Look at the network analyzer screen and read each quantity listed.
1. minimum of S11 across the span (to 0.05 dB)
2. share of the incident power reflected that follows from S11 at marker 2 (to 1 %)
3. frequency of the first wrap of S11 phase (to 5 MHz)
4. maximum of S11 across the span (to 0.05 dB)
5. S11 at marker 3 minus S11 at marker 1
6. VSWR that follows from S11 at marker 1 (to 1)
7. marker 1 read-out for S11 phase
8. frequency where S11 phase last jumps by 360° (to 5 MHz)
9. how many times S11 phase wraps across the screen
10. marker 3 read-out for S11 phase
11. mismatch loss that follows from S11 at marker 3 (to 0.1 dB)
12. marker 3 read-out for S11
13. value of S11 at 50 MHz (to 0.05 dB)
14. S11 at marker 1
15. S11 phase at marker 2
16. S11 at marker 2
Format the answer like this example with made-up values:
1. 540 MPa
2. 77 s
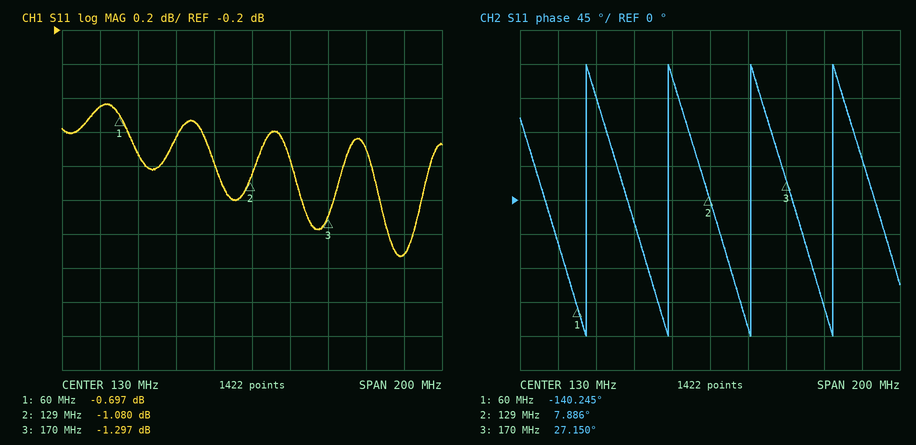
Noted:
1. -1.55 dB
2. 78 %
3. 65 MHz
4. -0.65 dB
5. -0.600 dB
6. 25
7. -140.245°
8. 195 MHz
9. 4
10. 27.150°
11. 5.9 dB
12. -1.297 dB
13. -0.65 dB
14. -0.697 dB
15. 7.886°
16. -1.080 dB
